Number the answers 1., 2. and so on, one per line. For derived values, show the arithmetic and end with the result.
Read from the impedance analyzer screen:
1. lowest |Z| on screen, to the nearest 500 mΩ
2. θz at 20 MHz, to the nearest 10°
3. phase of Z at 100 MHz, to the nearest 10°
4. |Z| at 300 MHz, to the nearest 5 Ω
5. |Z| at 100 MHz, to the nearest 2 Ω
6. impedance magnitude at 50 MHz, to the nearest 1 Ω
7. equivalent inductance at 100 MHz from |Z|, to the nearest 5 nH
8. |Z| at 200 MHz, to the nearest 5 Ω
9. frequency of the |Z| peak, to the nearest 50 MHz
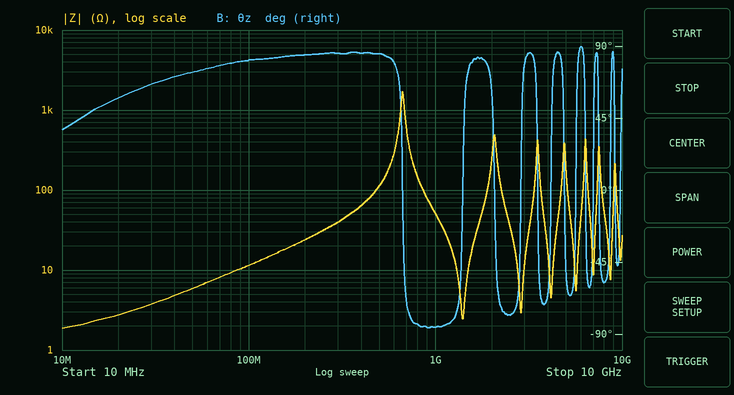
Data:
1. 2.0 Ω
2. 60°
3. 80°
4. 40 Ω
5. 12 Ω
6. 6 Ω
7. L = 12 Ω/(2π × 100 MHz) ≈ 19.1 nH, so 20 nH to the nearest 5 nH
8. 25 Ω
9. 650 MHz
